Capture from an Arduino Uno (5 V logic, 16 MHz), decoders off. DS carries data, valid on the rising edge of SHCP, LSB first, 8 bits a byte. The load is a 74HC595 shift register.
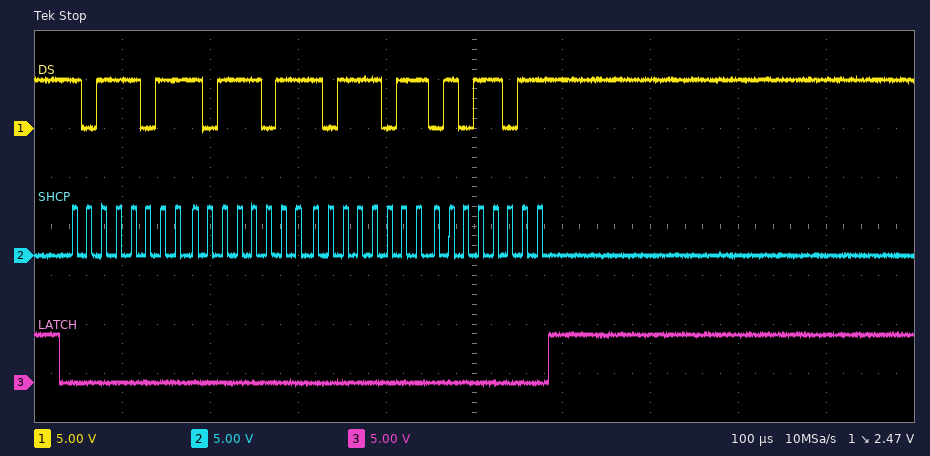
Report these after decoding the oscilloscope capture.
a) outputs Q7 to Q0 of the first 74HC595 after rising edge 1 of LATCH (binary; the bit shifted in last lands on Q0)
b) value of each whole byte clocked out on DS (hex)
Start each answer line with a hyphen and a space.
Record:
- 01011011
- DD DD DD DA
